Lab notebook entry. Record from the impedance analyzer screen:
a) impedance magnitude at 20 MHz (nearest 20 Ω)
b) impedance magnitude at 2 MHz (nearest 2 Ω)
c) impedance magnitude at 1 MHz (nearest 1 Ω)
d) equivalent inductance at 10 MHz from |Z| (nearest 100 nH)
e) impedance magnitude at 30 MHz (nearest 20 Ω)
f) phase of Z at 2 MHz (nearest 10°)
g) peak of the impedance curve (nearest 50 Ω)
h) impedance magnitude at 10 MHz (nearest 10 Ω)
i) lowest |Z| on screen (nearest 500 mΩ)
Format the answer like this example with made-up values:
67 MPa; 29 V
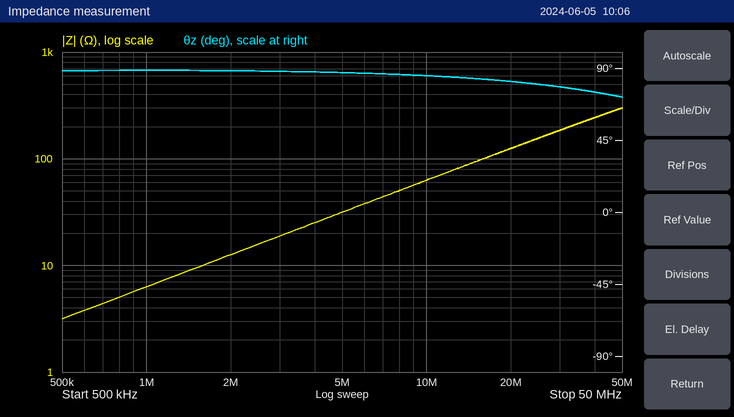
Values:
120 Ω; 12 Ω; 6 Ω; 1.0 µH; 180 Ω; 90°; 300 Ω; 60 Ω; 3.0 Ω
